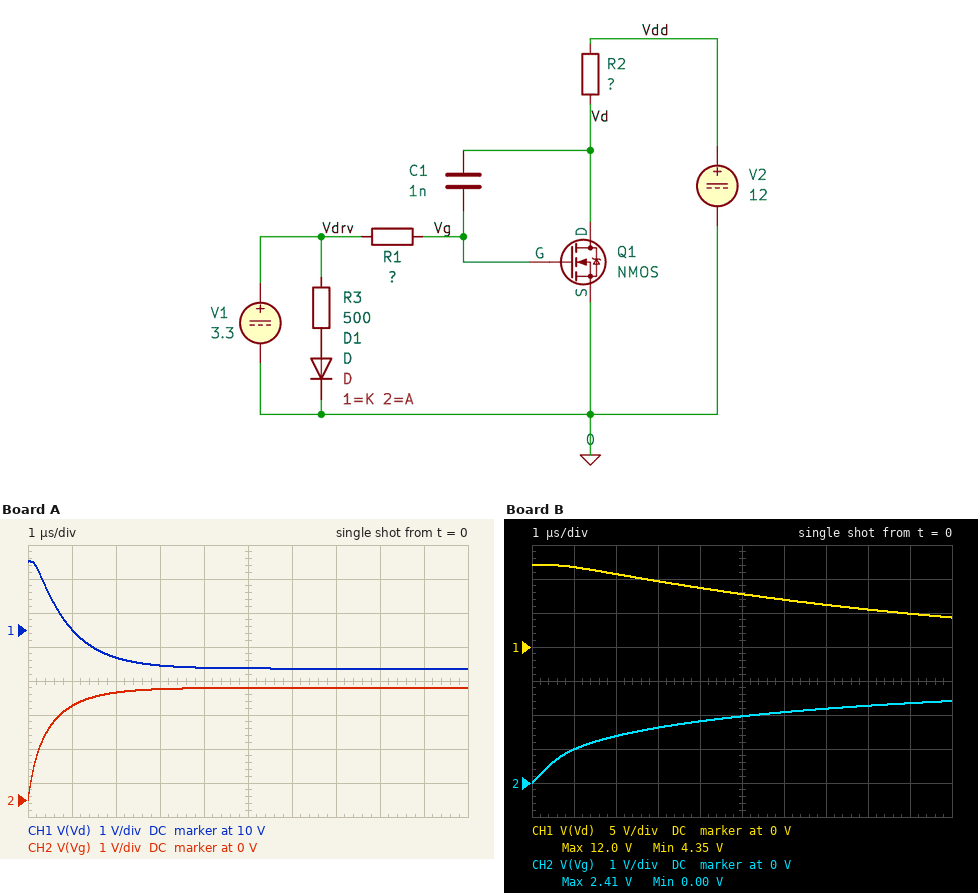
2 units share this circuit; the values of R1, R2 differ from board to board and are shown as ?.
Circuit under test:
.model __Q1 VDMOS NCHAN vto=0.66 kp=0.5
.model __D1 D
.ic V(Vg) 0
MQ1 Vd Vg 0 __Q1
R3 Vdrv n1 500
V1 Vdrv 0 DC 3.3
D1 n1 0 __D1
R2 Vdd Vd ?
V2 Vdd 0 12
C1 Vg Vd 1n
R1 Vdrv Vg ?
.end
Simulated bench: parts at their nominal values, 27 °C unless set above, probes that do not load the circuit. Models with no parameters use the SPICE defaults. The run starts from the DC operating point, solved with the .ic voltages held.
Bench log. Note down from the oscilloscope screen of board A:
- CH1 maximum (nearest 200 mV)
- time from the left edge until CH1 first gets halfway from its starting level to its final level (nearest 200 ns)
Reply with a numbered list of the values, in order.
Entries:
1. 12.0 V
2. 800 ns
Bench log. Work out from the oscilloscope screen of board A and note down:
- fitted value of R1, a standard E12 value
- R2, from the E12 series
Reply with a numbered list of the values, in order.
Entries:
1. 150 Ω
2. 1.8 Ω
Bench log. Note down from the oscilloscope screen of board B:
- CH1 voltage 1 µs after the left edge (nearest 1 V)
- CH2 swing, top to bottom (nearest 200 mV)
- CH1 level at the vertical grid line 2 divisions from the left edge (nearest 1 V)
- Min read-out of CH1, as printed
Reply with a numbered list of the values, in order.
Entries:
1. 12 V
2. 2.4 V
3. 11 V
4. 4.35 V
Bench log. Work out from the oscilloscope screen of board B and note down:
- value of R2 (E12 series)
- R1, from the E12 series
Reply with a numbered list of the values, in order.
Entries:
1. 10 Ω
2. 1 kΩ
